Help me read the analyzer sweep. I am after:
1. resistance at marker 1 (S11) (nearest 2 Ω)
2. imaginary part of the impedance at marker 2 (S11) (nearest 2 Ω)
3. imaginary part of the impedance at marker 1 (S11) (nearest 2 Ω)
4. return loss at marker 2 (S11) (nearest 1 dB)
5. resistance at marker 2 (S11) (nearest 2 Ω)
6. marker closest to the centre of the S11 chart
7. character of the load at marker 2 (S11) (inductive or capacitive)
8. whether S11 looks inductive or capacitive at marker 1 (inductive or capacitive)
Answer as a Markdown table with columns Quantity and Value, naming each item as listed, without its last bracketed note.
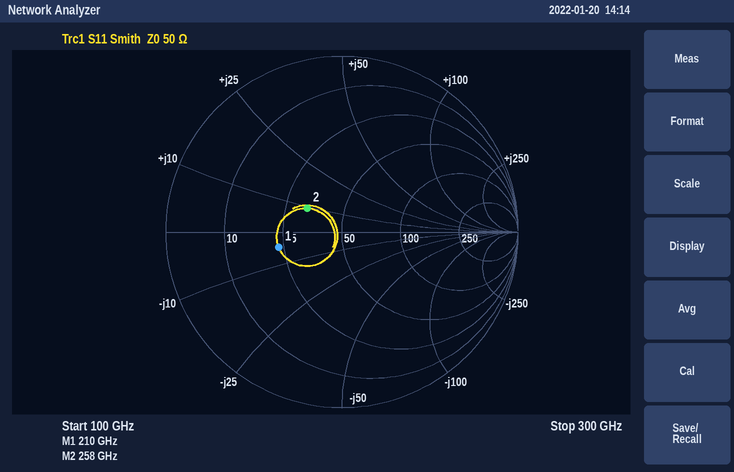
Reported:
| Quantity | Value |
|---|---|
| resistance at marker 1 (S11) | 24 Ω |
| imaginary part of the impedance at marker 2 (S11) | +10 Ω |
| imaginary part of the impedance at marker 1 (S11) | -4 Ω |
| return loss at marker 2 (S11) | 12 dB |
| resistance at marker 2 (S11) | 32 Ω |
| marker closest to the centre of the S11 chart | marker 2 |
| character of the load at marker 2 (S11) | inductive |
| whether S11 looks inductive or capacitive at marker 1 | capacitive |
